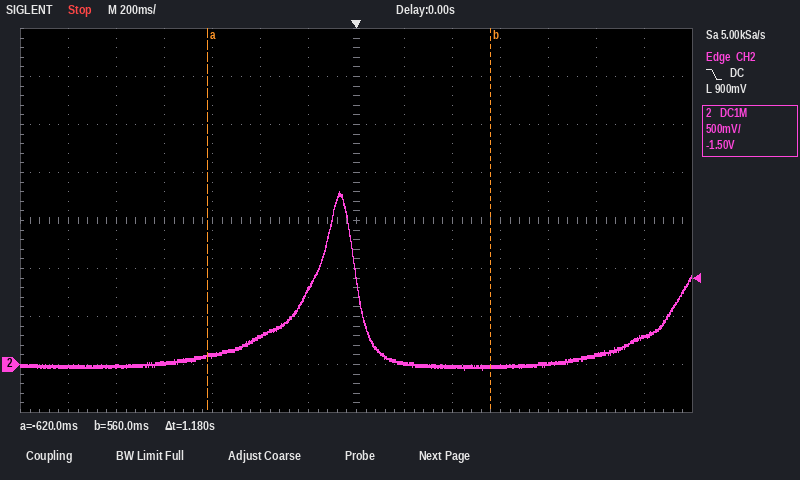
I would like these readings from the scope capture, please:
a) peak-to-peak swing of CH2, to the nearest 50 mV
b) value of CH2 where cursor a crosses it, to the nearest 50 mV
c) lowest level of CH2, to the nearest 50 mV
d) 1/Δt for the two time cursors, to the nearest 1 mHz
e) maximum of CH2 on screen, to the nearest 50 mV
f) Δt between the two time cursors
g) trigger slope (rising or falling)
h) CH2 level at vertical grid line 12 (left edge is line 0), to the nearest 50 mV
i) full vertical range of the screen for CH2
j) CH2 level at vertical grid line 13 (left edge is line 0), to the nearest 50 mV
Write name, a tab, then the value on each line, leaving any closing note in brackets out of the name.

peak-to-peak swing of CH2, to the nearest 50 mV	1.85 V
value of CH2 where cursor a crosses it, to the nearest 50 mV	100 mV
lowest level of CH2, to the nearest 50 mV	-50 mV
1/Δt for the two time cursors, to the nearest 1 mHz	847 mHz
maximum of CH2 on screen, to the nearest 50 mV	1.80 V
Δt between the two time cursors	1.18 s
trigger slope	falling
CH2 level at vertical grid line 12 (left edge is line 0), to the nearest 50 mV	100 mV
full vertical range of the screen for CH2	4 V
CH2 level at vertical grid line 13 (left edge is line 0), to the nearest 50 mV	300 mV
